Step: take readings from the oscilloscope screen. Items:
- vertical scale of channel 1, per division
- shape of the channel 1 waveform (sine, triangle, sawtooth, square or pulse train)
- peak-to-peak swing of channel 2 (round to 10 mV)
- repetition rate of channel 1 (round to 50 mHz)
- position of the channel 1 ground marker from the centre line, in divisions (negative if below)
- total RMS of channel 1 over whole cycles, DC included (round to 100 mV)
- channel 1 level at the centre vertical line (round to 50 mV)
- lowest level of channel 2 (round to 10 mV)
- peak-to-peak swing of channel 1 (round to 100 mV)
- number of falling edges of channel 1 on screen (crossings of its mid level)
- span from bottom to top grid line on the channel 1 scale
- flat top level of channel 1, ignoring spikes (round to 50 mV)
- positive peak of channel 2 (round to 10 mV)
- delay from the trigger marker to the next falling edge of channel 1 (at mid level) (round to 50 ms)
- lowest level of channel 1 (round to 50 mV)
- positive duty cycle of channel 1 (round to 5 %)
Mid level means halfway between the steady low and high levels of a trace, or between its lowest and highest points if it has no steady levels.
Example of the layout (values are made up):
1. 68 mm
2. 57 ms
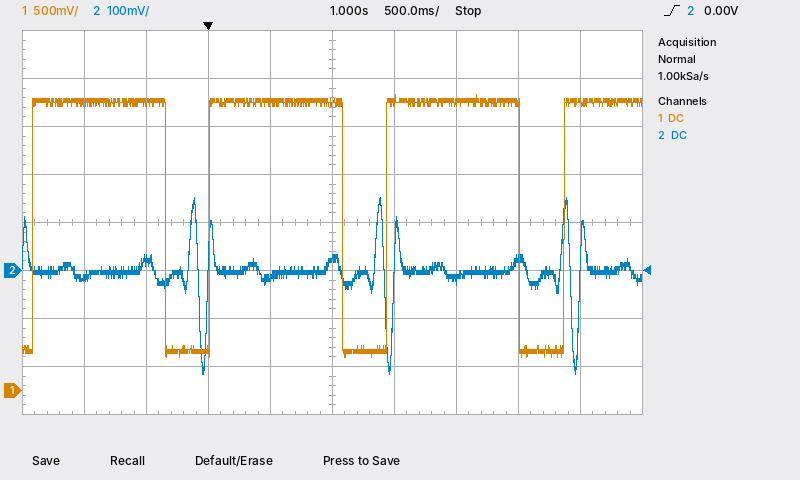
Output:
1. 500 mV
2. pulse train
3. 370 mV
4. 700 mHz
5. -3.5 div
6. 2.6 V
7. 3.00 V
8. -220 mV
9. 2.70 V
10. 3
11. 4 V
12. 3.00 V
13. 150 mV
14. 1.10 s
15. 350 mV
16. 75 %
